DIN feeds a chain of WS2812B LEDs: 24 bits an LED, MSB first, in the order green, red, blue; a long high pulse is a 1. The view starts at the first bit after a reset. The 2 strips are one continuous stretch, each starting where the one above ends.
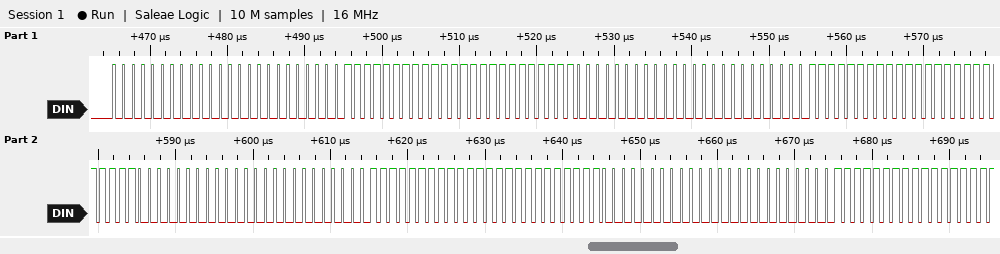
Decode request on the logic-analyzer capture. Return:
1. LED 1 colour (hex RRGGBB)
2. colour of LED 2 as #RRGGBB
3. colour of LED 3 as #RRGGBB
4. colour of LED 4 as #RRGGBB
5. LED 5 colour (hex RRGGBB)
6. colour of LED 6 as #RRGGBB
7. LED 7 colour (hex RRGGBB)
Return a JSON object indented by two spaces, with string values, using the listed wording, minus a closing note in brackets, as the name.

{
  "LED 1 colour": "#000000",
  "colour of LED 2 as #RRGGBB": "#FFFFFF",
  "colour of LED 3 as #RRGGBB": "#000000",
  "colour of LED 4 as #RRGGBB": "#FFFFFF",
  "LED 5 colour": "#000000",
  "colour of LED 6 as #RRGGBB": "#FFFFFF",
  "LED 7 colour": "#000000"
}
